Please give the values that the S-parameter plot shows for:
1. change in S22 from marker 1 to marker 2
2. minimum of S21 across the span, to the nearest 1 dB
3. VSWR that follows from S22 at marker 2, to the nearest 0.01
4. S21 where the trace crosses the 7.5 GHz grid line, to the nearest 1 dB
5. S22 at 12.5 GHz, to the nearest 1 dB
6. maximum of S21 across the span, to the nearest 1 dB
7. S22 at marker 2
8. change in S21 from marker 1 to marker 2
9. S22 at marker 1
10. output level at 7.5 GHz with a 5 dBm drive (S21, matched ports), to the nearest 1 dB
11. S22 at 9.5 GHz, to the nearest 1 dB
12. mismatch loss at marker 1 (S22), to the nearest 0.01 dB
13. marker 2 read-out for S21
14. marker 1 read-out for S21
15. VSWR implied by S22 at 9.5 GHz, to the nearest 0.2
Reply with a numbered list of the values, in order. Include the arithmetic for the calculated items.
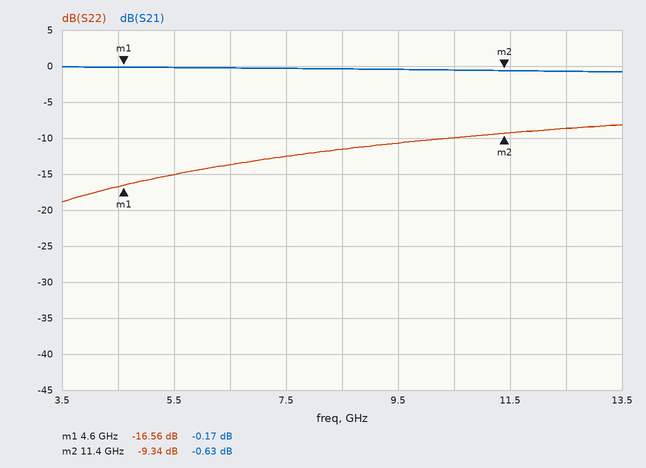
1. -9.34 − (-16.56) = 7.22 dB
2. -1 dB
3. (1 + 0.3412)/(1 − 0.3412) ≈ 2.04
4. 0 dB
5. -9 dB
6. 0 dB
7. -9.34 dB
8. -0.63 − (-0.17) = -0.46 dB
9. -16.56 dB
10. 5 dBm + (0 dB) = 5 dBm
11. -11 dB
12. −10 log10(1 − 10^(-16.56/10)) ≈ 0.10 dB
13. -0.63 dB
14. -0.17 dB
15. |Γ| = 10^(-11/20) = 0.2818; VSWR = (1 + 0.2818)/(1 − 0.2818) ≈ 1.8
